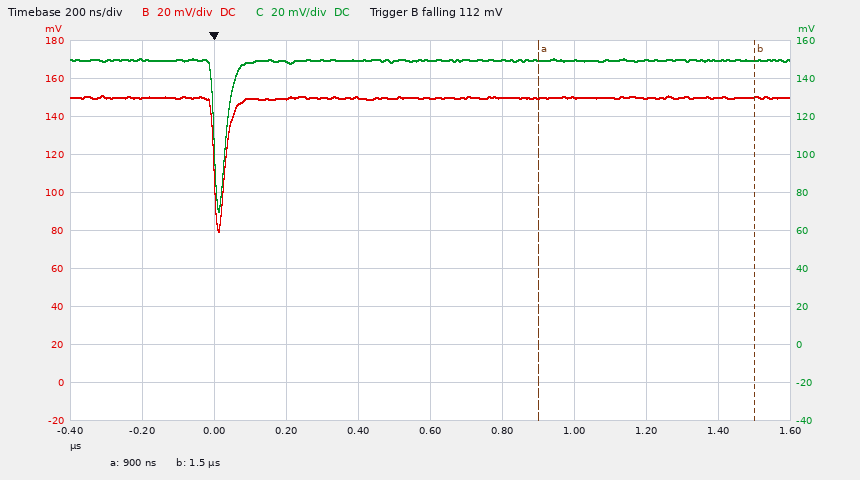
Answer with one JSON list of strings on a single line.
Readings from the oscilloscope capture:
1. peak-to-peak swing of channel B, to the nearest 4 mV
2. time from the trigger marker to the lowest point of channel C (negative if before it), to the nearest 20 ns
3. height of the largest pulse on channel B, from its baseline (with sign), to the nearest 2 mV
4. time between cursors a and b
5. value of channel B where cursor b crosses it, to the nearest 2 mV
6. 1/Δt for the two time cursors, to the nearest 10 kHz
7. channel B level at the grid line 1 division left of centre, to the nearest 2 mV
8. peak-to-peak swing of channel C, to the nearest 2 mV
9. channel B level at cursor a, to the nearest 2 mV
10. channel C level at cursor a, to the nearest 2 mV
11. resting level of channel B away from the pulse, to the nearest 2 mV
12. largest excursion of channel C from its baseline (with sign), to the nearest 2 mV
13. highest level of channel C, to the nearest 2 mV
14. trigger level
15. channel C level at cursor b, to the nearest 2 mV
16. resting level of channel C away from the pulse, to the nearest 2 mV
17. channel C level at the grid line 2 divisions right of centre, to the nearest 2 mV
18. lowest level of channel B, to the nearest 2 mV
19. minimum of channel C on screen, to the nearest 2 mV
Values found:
["72 mV", "+20 ns", "-70 mV", "600 ns", "150 mV", "1.67 MHz", "150 mV", "80 mV", "150 mV", "150 mV", "150 mV", "-80 mV", "150 mV", "112 mV", "150 mV", "150 mV", "150 mV", "80 mV", "70 mV"]
